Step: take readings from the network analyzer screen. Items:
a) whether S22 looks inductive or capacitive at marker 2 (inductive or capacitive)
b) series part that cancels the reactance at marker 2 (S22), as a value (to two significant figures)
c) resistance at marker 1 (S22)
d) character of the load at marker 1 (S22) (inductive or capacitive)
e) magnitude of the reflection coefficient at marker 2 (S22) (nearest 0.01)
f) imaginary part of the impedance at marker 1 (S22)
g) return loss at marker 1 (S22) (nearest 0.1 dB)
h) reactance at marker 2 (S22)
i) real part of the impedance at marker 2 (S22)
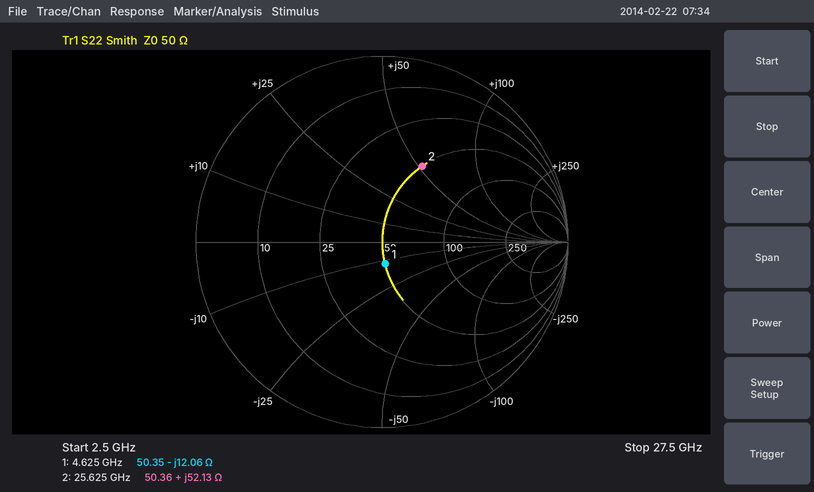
inductive
120 fF
50.35 Ω
capacitive
0.46
-12.06 Ω
18.5 dB
+52.13 Ω
50.36 Ω
